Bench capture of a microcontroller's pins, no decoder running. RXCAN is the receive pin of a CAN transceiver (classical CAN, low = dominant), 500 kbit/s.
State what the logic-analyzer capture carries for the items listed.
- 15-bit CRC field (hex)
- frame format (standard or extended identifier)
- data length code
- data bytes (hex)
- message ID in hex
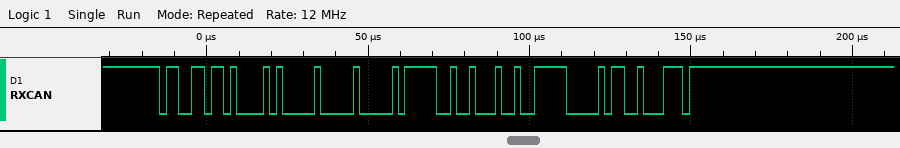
0x0323
standard
5
00 00 FA 44 9F
0x66D
